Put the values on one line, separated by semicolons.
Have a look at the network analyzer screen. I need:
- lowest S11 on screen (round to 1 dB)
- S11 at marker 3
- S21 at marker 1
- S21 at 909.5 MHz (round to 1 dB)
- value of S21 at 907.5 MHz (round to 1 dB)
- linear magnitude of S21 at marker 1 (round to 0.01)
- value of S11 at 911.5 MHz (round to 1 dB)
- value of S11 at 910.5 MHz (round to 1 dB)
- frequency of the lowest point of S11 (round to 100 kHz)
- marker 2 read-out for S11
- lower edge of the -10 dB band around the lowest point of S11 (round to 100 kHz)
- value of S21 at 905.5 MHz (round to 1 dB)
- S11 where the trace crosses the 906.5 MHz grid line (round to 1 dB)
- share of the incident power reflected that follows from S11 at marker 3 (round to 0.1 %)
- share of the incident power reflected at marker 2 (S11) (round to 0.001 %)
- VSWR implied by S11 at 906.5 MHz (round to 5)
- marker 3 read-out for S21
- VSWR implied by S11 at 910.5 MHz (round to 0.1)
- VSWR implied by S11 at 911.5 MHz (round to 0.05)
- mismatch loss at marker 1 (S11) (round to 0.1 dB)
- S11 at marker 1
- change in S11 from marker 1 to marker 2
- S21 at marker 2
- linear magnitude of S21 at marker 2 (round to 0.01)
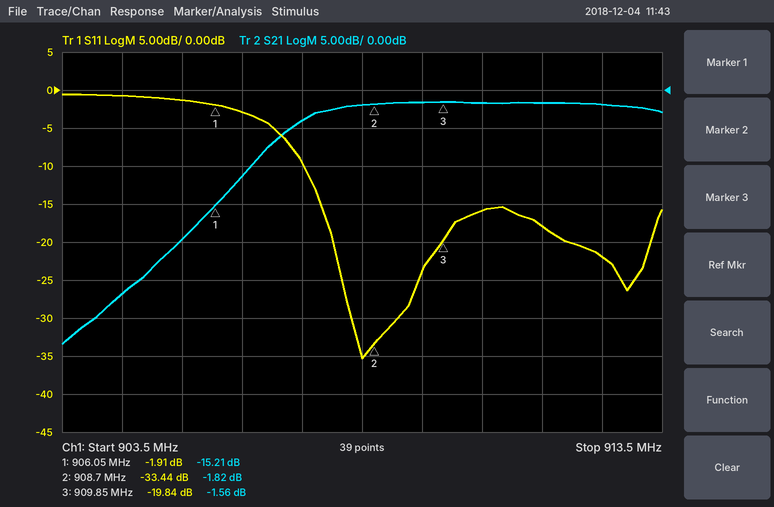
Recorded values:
-35 dB; -19.84 dB; -15.21 dB; -2 dB; -4 dB; 0.17; -18 dB; -16 dB; 908.5 MHz; -33.44 dB; 907.5 MHz; -20 dB; -3 dB; 1.0 %; 0.045 %; 5; -1.56 dB; 1.4; 1.30; 4.5 dB; -1.91 dB; -31.53 dB; -1.82 dB; 0.81
